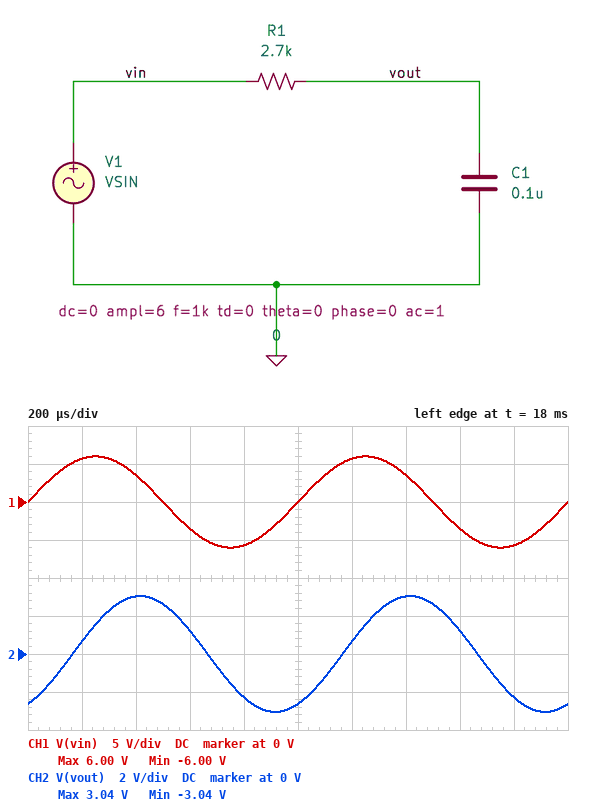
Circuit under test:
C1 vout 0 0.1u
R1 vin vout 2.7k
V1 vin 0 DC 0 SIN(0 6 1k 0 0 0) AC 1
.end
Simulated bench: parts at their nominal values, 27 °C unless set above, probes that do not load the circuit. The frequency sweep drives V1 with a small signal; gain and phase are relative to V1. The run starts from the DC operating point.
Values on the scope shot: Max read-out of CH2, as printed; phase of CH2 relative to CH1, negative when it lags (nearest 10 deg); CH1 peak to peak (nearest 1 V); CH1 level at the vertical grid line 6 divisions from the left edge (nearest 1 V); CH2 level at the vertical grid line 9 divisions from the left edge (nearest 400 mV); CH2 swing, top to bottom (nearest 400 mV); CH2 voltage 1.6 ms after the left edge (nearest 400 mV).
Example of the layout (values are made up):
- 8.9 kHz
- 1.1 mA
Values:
- 3.04 V
- -60 deg
- 12 V
- 6 V
- -2.4 V
- 6.0 V
- 1.2 V
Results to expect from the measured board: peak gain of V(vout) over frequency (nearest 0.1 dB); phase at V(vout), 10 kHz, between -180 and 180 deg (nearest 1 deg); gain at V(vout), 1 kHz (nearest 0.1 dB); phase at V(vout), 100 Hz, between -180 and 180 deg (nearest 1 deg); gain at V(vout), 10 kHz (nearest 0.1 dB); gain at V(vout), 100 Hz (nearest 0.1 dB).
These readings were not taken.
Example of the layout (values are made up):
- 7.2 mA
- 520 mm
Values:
- 0 dB
- -87 deg
- -5.9 dB
- -10 deg
- -24.6 dB
- -0.1 dB
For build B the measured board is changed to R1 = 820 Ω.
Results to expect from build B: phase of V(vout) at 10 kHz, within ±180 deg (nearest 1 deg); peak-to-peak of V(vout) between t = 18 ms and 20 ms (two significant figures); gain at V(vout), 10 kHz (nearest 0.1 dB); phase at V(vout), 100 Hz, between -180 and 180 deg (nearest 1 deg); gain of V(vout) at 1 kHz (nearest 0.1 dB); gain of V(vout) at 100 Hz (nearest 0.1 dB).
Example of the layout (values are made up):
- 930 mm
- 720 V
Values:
- -79 deg
- 11 V
- -14.4 dB
- -3 deg
- -1.0 dB
- 0 dB
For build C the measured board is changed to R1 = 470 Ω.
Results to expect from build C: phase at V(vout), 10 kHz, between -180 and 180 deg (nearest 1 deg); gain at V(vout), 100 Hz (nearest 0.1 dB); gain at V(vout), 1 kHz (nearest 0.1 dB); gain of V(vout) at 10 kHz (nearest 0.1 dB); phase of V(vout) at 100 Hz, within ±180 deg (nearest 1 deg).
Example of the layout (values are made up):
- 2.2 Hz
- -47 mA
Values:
- -71 deg
- 0 dB
- -0.4 dB
- -9.9 dB
- -2 deg
